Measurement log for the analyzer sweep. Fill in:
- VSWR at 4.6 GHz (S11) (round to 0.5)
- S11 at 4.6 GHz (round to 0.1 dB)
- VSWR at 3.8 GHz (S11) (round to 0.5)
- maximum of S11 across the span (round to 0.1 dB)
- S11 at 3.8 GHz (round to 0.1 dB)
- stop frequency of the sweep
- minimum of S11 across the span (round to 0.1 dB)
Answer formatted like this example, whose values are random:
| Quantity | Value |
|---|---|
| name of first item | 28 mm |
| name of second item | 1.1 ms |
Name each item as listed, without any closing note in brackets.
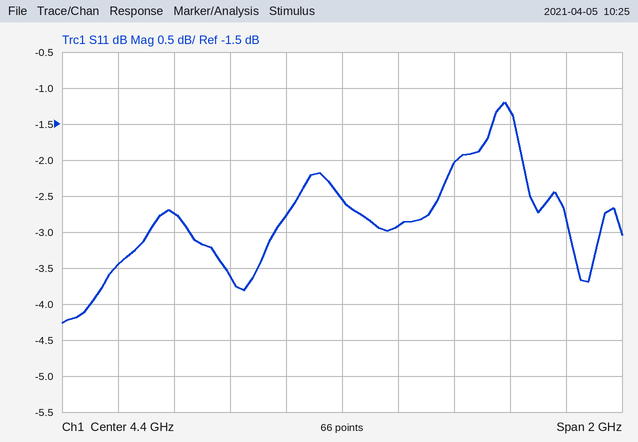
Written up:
| Quantity | Value |
|---|---|
| VSWR at 4.6 GHz (S11) | 6.0 |
| S11 at 4.6 GHz | -2.9 dB |
| VSWR at 3.8 GHz (S11) | 6.5 |
| maximum of S11 across the span | -1.2 dB |
| S11 at 3.8 GHz | -2.7 dB |
| stop frequency of the sweep | 5.4 GHz |
| minimum of S11 across the span | -4.3 dB |
